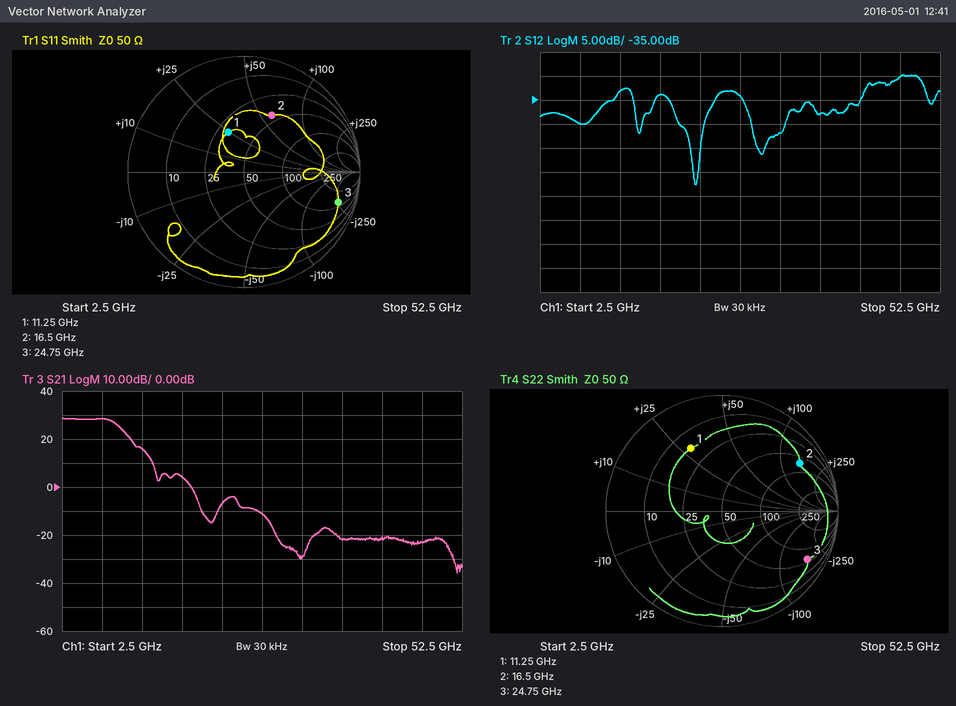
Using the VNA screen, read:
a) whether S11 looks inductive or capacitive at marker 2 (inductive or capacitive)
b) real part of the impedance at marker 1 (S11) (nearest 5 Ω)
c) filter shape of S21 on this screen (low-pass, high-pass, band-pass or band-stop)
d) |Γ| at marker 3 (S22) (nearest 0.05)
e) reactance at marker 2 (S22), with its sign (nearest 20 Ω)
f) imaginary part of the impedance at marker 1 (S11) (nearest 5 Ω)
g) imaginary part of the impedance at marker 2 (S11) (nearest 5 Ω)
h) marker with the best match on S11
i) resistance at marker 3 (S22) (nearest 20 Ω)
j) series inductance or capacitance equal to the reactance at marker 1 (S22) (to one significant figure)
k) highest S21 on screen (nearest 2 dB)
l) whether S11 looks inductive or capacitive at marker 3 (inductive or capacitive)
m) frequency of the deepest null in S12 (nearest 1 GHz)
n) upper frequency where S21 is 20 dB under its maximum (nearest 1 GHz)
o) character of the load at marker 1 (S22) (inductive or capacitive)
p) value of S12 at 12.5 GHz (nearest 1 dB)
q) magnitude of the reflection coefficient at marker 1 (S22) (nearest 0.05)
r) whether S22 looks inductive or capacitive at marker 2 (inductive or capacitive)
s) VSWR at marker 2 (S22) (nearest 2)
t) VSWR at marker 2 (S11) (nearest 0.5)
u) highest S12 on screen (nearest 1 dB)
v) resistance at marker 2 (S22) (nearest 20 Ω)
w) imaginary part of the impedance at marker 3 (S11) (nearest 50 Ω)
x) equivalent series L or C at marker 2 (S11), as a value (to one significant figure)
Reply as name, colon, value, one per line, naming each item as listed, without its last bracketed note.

whether S11 looks inductive or capacitive at marker 2: inductive
real part of the impedance at marker 1 (S11): 30 Ω
filter shape of S21 on this screen: low-pass
|Γ| at marker 3 (S22): 0.85
reactance at marker 2 (S22), with its sign: +140 Ω
imaginary part of the impedance at marker 1 (S11): +25 Ω
imaginary part of the impedance at marker 2 (S11): +60 Ω
marker with the best match on S11: marker 1
resistance at marker 3 (S22): 60 Ω
series inductance or capacitance equal to the reactance at marker 1 (S22): 400 pH
highest S21 on screen: 28 dB
whether S11 looks inductive or capacitive at marker 3: capacitive
frequency of the deepest null in S12: 22 GHz
upper frequency where S21 is 20 dB under its maximum: 14 GHz
character of the load at marker 1 (S22): inductive
value of S12 at 12.5 GHz: -33 dB
magnitude of the reflection coefficient at marker 1 (S22): 0.60
whether S22 looks inductive or capacitive at marker 2: inductive
VSWR at marker 2 (S22): 8
VSWR at marker 2 (S11): 3.5
highest S12 on screen: -30 dB
resistance at marker 2 (S22): 60 Ω
imaginary part of the impedance at marker 3 (S11): -250 Ω
equivalent series L or C at marker 2 (S11), as a value: 600 pH
